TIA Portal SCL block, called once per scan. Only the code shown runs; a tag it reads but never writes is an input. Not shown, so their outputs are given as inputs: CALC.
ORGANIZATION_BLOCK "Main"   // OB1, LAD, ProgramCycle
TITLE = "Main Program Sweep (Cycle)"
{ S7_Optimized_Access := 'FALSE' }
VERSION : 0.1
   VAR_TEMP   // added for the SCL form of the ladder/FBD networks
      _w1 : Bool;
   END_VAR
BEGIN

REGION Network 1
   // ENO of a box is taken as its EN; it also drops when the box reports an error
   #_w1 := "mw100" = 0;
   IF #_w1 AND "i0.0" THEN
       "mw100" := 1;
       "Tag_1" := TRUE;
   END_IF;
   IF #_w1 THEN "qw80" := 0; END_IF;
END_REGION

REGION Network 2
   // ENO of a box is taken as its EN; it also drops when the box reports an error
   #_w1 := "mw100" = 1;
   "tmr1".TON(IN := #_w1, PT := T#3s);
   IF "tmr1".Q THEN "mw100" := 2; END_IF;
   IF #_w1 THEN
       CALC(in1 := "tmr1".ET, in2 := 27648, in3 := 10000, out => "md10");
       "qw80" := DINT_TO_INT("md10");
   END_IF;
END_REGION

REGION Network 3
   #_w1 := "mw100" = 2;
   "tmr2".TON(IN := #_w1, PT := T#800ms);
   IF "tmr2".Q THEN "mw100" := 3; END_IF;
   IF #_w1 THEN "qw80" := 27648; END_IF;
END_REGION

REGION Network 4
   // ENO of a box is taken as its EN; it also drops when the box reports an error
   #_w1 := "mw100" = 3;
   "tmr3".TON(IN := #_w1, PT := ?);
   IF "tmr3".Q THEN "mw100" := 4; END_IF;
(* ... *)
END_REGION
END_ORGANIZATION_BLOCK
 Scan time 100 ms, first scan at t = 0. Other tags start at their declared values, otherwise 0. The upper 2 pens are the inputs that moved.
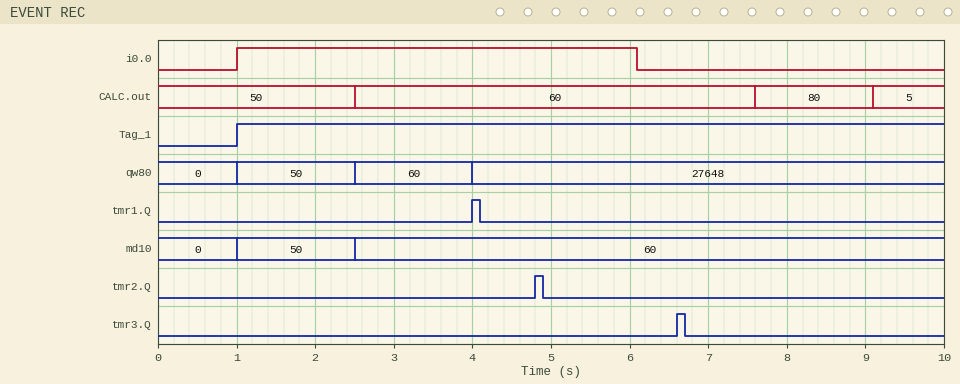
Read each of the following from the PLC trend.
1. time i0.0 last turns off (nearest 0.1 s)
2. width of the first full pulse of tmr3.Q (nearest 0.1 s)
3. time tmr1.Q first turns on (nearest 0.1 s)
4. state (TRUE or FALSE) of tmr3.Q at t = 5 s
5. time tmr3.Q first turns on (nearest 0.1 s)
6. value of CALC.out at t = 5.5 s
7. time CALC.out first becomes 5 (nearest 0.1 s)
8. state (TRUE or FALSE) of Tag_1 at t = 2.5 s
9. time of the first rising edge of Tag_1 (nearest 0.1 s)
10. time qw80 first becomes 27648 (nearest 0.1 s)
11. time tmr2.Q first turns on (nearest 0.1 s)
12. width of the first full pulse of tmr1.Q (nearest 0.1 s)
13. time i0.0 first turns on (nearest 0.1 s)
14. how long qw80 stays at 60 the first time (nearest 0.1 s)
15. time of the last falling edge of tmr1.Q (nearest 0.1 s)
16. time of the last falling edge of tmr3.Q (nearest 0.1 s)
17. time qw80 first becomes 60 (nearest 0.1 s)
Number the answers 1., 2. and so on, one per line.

1. 6.1 s
2. 0.1 s
3. 4.0 s
4. FALSE
5. 6.6 s
6. 60
7. 9.1 s
8. TRUE
9. 1.0 s
10. 4.0 s
11. 4.8 s
12. 0.1 s
13. 1.0 s
14. 1.5 s
15. 4.1 s
16. 6.7 s
17. 2.5 s
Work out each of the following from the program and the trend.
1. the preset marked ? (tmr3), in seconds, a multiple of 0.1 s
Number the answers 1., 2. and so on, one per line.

1. 1.8 s
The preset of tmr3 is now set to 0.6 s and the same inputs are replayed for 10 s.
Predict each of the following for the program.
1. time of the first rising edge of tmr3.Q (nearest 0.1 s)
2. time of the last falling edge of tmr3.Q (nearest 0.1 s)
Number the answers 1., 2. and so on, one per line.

1. 5.4 s
2. 5.5 s
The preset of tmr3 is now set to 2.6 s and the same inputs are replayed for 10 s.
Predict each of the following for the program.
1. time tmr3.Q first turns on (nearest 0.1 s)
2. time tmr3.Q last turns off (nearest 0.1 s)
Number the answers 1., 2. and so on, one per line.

1. 7.4 s
2. 7.5 s
